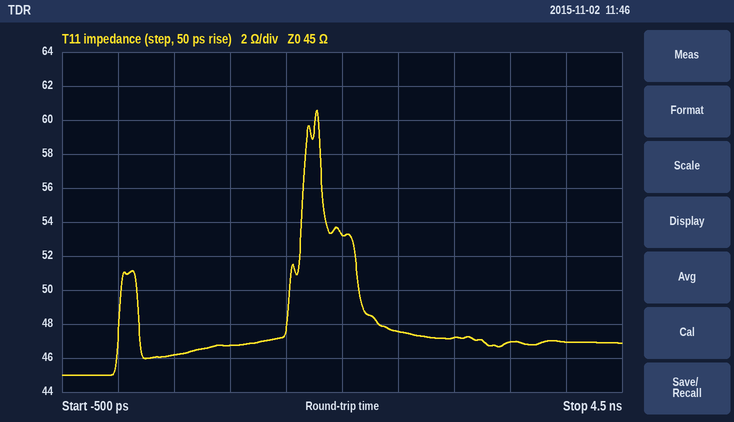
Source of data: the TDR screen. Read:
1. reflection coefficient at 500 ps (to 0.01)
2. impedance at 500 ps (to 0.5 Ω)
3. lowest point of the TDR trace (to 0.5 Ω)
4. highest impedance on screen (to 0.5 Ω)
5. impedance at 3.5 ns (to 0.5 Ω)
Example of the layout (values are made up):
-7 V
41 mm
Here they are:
+0.01
46.0 Ω
45.0 Ω
60.5 Ω
47.0 Ω
